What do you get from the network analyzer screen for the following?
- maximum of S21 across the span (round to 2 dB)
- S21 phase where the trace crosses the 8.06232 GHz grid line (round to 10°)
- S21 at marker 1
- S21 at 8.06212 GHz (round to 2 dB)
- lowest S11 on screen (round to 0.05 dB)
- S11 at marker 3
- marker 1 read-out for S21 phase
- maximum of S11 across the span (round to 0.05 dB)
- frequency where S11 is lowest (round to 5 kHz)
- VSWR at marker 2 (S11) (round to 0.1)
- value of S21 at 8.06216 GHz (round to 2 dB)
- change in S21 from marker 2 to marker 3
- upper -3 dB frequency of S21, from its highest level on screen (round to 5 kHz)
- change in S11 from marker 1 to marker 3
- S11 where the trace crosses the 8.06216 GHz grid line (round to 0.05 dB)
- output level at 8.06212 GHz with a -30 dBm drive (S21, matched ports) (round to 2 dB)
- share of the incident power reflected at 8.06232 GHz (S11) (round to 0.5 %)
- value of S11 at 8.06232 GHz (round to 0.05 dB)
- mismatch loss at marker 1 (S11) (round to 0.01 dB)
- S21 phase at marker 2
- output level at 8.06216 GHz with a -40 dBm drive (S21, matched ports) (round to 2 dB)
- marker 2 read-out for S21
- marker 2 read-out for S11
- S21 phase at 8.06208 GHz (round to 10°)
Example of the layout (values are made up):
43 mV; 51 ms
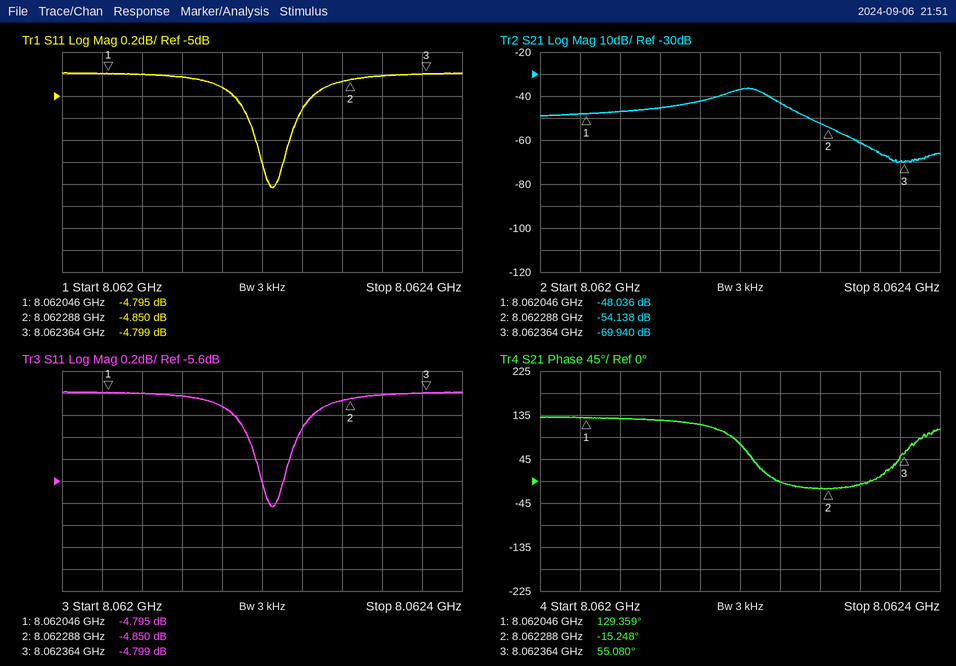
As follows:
-36 dB; -10°; -48.036 dB; -46 dB; -5.85 dB; -4.799 dB; 129.359°; -4.80 dB; 8.062210 GHz; 3.7; -42 dB; -15.802 dB; 8.062225 GHz; -0.004 dB; -4.90 dB; -76 dBm; 33.0 %; -4.80 dB; 1.75 dB; -15.248°; -82 dBm; -54.138 dB; -4.850 dB; 130°
